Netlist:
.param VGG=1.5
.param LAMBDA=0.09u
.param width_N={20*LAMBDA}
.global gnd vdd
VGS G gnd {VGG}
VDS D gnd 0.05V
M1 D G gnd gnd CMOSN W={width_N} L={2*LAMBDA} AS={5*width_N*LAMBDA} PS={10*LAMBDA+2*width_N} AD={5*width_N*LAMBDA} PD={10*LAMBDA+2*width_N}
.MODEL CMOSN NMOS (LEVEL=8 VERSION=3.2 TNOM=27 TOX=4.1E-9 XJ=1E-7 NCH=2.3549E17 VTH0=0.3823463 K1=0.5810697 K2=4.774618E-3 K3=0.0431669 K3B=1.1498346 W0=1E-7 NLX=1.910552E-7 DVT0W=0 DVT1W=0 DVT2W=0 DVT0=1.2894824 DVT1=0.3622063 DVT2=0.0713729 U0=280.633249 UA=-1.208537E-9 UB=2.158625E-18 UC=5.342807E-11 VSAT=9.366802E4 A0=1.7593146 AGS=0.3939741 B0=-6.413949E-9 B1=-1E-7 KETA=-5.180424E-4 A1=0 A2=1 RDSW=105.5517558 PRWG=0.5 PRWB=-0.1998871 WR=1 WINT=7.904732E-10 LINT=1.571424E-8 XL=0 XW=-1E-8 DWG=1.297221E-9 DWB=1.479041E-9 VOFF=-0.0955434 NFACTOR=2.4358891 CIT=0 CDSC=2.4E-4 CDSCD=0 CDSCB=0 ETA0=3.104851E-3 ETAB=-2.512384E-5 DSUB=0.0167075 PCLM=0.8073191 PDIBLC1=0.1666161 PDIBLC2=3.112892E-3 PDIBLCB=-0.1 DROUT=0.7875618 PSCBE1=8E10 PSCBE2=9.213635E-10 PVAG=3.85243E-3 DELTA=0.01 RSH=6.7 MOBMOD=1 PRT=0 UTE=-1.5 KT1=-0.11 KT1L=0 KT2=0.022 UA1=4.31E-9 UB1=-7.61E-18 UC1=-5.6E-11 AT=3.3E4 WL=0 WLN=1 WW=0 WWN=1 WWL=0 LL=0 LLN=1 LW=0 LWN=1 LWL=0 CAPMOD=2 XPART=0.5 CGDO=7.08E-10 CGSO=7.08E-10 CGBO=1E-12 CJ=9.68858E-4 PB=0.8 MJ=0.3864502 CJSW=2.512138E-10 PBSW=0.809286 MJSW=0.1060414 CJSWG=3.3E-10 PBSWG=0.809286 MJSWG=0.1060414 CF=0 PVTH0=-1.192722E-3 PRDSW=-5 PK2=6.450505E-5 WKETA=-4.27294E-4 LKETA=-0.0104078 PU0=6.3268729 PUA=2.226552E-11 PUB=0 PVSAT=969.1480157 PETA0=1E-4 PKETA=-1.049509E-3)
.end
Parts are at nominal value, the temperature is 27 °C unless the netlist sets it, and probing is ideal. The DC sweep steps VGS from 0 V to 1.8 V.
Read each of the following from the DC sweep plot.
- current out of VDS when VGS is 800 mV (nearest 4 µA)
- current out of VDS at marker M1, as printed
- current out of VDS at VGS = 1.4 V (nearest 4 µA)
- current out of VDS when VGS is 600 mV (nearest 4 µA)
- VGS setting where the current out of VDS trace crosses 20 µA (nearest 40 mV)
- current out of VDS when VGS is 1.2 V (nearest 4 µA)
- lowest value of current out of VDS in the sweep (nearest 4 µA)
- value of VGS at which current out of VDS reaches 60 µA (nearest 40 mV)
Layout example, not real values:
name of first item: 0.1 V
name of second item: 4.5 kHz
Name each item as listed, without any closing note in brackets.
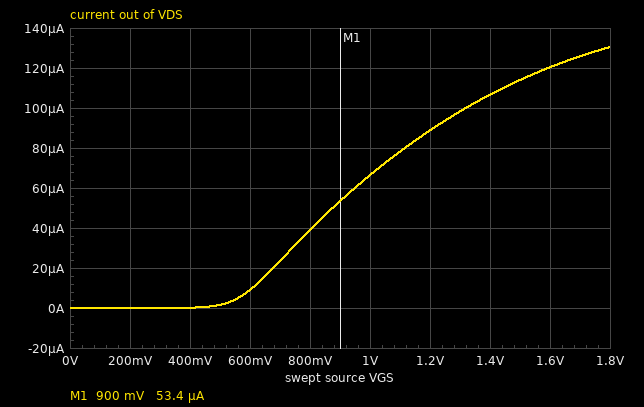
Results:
current out of VDS when VGS is 800 mV: 40 µA
current out of VDS at marker M1, as printed: 53.4 µA
current out of VDS at VGS = 1.4 V: 108 µA
current out of VDS when VGS is 600 mV: 8 µA
VGS setting where the current out of VDS trace crosses 20 µA: 680 mV
current out of VDS when VGS is 1.2 V: 88 µA
lowest value of current out of VDS in the sweep: 0 A
value of VGS at which current out of VDS reaches 60 µA: 960 mV
